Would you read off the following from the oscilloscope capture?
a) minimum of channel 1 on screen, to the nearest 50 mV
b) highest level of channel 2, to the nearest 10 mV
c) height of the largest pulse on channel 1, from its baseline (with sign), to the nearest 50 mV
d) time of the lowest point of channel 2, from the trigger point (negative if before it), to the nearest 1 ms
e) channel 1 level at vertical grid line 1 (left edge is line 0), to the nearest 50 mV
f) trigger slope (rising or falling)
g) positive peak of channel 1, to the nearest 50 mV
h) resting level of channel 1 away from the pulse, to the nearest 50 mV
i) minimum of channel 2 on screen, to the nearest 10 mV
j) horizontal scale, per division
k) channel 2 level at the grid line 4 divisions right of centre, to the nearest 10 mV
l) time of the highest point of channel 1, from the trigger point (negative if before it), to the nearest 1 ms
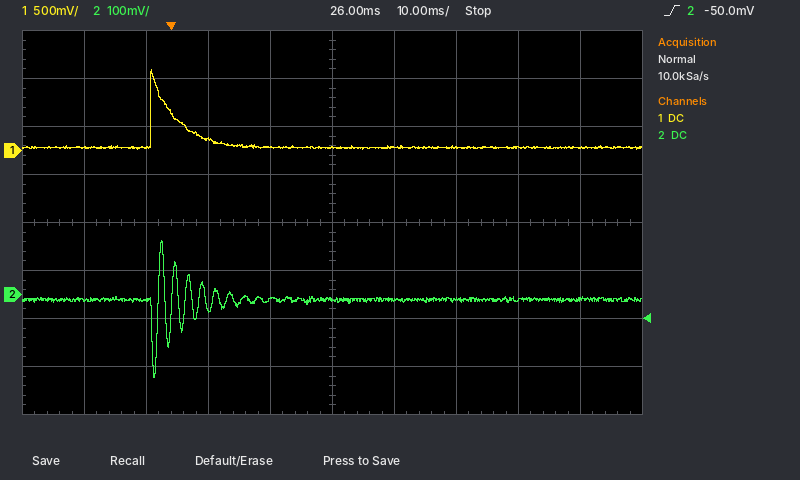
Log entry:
0 mV
110 mV
+800 mV
-3 ms
50 mV
rising
850 mV
50 mV
-170 mV
10 ms
-10 mV
-3 ms
